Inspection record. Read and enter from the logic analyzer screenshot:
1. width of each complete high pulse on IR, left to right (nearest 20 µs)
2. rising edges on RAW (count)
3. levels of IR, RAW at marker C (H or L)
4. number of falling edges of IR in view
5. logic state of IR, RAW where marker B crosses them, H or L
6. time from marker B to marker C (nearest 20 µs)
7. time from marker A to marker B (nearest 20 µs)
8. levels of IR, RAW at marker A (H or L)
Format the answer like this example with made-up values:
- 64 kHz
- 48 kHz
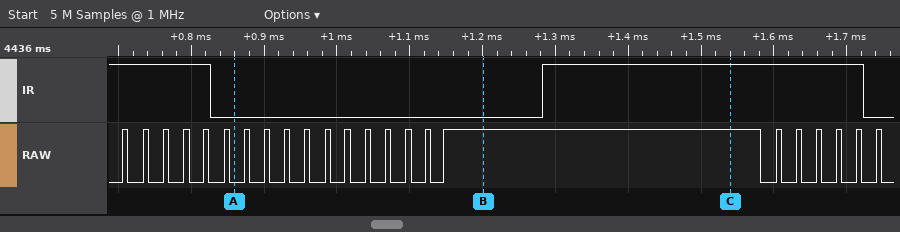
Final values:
- 440 µs
- 23
- IR=H, RAW=H
- 2
- IR=L, RAW=H
- 340 µs
- 340 µs
- IR=L, RAW=L
